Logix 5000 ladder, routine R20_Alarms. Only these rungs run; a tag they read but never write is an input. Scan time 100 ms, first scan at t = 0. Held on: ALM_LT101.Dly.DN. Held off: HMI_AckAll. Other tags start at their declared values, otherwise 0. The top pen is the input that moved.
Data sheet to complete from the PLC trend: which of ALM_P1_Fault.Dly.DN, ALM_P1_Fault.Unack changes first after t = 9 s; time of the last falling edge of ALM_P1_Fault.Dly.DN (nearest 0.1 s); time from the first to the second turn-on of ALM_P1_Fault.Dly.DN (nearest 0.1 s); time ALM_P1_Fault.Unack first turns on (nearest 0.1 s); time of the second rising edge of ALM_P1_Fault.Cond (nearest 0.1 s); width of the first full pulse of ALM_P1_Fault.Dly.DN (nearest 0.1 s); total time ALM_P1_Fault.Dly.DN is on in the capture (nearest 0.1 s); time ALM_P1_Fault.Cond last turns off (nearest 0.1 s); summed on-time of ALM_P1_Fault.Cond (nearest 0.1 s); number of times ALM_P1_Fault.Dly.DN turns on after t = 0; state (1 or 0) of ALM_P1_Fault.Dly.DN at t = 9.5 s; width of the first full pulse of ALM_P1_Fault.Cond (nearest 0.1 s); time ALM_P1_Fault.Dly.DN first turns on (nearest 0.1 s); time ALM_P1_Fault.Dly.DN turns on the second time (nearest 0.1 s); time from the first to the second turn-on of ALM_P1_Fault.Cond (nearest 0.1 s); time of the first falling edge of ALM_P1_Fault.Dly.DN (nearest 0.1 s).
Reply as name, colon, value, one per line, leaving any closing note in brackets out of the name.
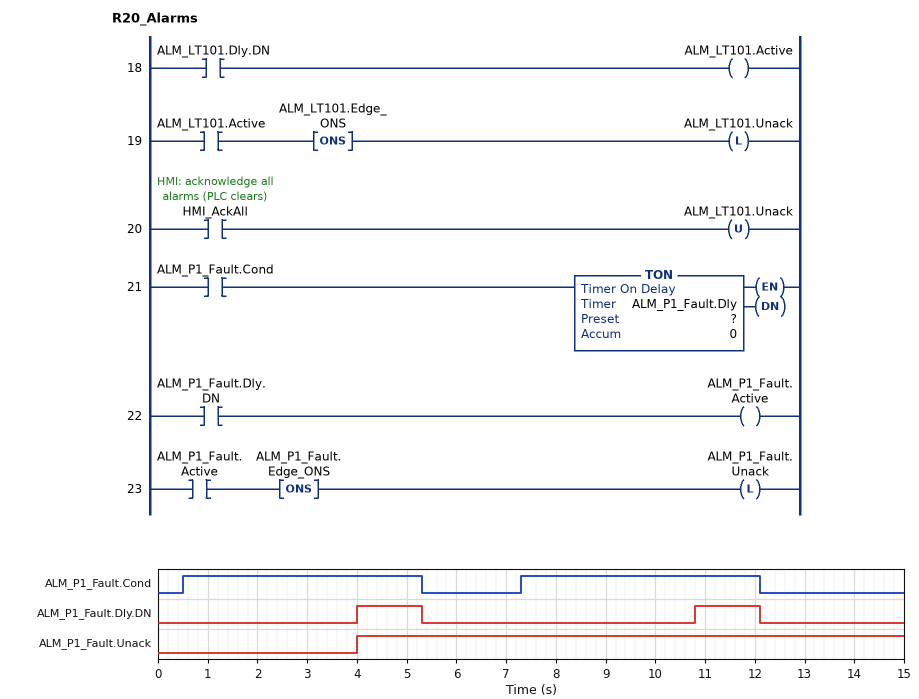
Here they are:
which of ALM_P1_Fault.Dly.DN, ALM_P1_Fault.Unack changes first after t = 9 s: ALM_P1_Fault.Dly.DN
time of the last falling edge of ALM_P1_Fault.Dly.DN: 12.1 s
time from the first to the second turn-on of ALM_P1_Fault.Dly.DN: 6.8 s
time ALM_P1_Fault.Unack first turns on: 4.0 s
time of the second rising edge of ALM_P1_Fault.Cond: 7.3 s
width of the first full pulse of ALM_P1_Fault.Dly.DN: 1.3 s
total time ALM_P1_Fault.Dly.DN is on in the capture: 2.6 s
time ALM_P1_Fault.Cond last turns off: 12.1 s
summed on-time of ALM_P1_Fault.Cond: 9.6 s
number of times ALM_P1_Fault.Dly.DN turns on after t = 0: 2
state (1 or 0) of ALM_P1_Fault.Dly.DN at t = 9.5 s: 0
width of the first full pulse of ALM_P1_Fault.Cond: 4.8 s
time ALM_P1_Fault.Dly.DN first turns on: 4.0 s
time ALM_P1_Fault.Dly.DN turns on the second time: 10.8 s
time from the first to the second turn-on of ALM_P1_Fault.Cond: 6.8 s
time of the first falling edge of ALM_P1_Fault.Dly.DN: 5.3 s
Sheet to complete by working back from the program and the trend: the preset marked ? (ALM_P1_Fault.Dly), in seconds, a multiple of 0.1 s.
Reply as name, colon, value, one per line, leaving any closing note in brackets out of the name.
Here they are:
the preset marked ? (ALM_P1_Fault.Dly), in seconds, a multiple of 0.1 s: 3.5 s
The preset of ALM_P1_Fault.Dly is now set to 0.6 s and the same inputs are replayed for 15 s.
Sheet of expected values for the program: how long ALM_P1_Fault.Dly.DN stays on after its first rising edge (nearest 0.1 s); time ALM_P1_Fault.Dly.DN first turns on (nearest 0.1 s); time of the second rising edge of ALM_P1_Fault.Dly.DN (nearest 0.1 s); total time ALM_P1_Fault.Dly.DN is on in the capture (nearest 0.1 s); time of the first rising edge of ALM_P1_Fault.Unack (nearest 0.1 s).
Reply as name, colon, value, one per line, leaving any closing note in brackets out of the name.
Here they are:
how long ALM_P1_Fault.Dly.DN stays on after its first rising edge: 4.2 s
time ALM_P1_Fault.Dly.DN first turns on: 1.1 s
time of the second rising edge of ALM_P1_Fault.Dly.DN: 7.9 s
total time ALM_P1_Fault.Dly.DN is on in the capture: 8.4 s
time of the first rising edge of ALM_P1_Fault.Unack: 1.1 s
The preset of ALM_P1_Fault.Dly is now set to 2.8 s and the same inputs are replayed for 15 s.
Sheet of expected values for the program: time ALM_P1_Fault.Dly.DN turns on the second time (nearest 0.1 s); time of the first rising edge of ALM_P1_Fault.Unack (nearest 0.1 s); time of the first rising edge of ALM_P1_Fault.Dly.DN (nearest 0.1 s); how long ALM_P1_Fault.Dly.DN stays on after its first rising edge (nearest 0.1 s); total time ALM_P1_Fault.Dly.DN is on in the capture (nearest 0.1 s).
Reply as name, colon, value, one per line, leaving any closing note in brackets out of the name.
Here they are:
time ALM_P1_Fault.Dly.DN turns on the second time: 10.1 s
time of the first rising edge of ALM_P1_Fault.Unack: 3.3 s
time of the first rising edge of ALM_P1_Fault.Dly.DN: 3.3 s
how long ALM_P1_Fault.Dly.DN stays on after its first rising edge: 2.0 s
total time ALM_P1_Fault.Dly.DN is on in the capture: 4.0 s
